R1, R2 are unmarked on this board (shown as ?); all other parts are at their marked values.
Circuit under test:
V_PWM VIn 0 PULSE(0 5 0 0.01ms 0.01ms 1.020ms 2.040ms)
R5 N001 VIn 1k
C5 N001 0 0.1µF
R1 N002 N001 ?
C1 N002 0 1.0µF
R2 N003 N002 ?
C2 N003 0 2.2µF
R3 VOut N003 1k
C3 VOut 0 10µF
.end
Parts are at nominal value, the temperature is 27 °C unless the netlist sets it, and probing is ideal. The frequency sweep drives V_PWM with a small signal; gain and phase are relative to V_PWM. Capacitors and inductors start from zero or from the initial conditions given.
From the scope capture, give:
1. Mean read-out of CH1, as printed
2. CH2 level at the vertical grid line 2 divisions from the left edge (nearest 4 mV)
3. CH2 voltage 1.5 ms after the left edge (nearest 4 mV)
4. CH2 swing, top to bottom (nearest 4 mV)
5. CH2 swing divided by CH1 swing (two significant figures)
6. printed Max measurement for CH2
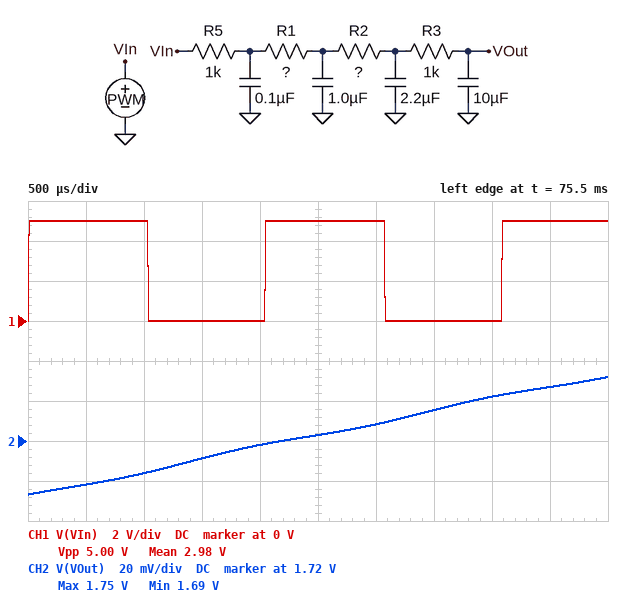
2.98 V
1.704 V
1.712 V
60 mV
0.012
1.75 V
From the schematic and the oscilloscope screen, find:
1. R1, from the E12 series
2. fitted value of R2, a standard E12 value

390 Ω
3.3 kΩ
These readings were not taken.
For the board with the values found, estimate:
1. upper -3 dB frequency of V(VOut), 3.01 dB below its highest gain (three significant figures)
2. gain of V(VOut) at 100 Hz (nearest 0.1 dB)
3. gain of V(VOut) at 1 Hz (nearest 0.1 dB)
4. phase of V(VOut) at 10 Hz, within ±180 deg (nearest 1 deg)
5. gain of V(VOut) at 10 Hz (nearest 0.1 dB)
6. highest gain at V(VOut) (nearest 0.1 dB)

2.41 Hz
-37.0 dB
-0.7 dB
-86 deg
-12.7 dB
0 dB
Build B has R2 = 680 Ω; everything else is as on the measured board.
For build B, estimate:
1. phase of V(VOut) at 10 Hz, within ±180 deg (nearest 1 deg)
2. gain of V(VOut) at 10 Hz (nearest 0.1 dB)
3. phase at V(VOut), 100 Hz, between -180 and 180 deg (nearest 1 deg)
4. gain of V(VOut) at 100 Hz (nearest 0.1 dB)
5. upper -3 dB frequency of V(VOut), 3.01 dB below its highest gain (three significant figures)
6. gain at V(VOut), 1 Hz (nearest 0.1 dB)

-73 deg
-7.6 dB
-148 deg
-30.3 dB
4.58 Hz
-0.2 dB
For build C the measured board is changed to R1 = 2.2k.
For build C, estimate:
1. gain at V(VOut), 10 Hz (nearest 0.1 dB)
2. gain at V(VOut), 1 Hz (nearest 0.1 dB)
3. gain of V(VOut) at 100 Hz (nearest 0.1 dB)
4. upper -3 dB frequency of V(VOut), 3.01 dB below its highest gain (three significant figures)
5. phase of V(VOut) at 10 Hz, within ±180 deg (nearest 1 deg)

-15.2 dB
-1.2 dB
-41.6 dB
1.78 Hz
-92 deg
